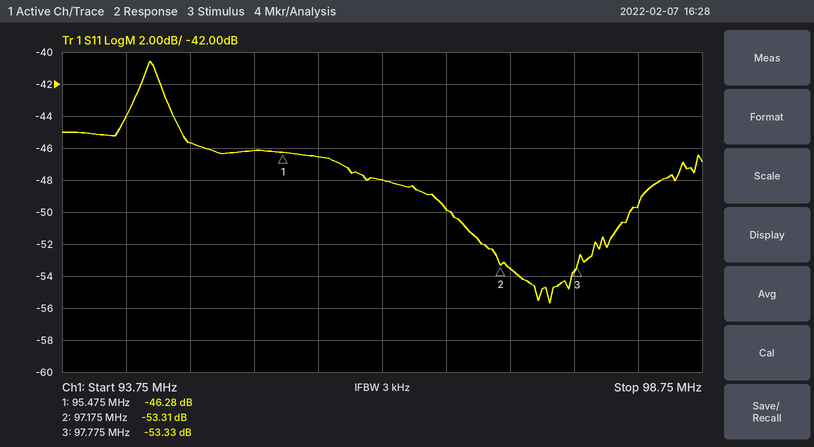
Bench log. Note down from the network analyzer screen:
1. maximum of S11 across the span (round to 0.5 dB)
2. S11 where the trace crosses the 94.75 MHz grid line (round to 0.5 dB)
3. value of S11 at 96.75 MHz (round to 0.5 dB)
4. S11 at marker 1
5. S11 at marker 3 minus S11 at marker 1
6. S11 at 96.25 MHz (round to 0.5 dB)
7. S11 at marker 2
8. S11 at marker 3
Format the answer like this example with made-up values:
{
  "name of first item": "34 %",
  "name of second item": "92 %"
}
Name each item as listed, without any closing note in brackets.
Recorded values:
{
  "maximum of S11 across the span": "-40.5 dB",
  "S11 where the trace crosses the 94.75 MHz grid line": "-45.5 dB",
  "value of S11 at 96.75 MHz": "-50.0 dB",
  "S11 at marker 1": "-46.28 dB",
  "S11 at marker 3 minus S11 at marker 1": "-7.05 dB",
  "S11 at 96.25 MHz": "-48.0 dB",
  "S11 at marker 2": "-53.31 dB",
  "S11 at marker 3": "-53.33 dB"
}
